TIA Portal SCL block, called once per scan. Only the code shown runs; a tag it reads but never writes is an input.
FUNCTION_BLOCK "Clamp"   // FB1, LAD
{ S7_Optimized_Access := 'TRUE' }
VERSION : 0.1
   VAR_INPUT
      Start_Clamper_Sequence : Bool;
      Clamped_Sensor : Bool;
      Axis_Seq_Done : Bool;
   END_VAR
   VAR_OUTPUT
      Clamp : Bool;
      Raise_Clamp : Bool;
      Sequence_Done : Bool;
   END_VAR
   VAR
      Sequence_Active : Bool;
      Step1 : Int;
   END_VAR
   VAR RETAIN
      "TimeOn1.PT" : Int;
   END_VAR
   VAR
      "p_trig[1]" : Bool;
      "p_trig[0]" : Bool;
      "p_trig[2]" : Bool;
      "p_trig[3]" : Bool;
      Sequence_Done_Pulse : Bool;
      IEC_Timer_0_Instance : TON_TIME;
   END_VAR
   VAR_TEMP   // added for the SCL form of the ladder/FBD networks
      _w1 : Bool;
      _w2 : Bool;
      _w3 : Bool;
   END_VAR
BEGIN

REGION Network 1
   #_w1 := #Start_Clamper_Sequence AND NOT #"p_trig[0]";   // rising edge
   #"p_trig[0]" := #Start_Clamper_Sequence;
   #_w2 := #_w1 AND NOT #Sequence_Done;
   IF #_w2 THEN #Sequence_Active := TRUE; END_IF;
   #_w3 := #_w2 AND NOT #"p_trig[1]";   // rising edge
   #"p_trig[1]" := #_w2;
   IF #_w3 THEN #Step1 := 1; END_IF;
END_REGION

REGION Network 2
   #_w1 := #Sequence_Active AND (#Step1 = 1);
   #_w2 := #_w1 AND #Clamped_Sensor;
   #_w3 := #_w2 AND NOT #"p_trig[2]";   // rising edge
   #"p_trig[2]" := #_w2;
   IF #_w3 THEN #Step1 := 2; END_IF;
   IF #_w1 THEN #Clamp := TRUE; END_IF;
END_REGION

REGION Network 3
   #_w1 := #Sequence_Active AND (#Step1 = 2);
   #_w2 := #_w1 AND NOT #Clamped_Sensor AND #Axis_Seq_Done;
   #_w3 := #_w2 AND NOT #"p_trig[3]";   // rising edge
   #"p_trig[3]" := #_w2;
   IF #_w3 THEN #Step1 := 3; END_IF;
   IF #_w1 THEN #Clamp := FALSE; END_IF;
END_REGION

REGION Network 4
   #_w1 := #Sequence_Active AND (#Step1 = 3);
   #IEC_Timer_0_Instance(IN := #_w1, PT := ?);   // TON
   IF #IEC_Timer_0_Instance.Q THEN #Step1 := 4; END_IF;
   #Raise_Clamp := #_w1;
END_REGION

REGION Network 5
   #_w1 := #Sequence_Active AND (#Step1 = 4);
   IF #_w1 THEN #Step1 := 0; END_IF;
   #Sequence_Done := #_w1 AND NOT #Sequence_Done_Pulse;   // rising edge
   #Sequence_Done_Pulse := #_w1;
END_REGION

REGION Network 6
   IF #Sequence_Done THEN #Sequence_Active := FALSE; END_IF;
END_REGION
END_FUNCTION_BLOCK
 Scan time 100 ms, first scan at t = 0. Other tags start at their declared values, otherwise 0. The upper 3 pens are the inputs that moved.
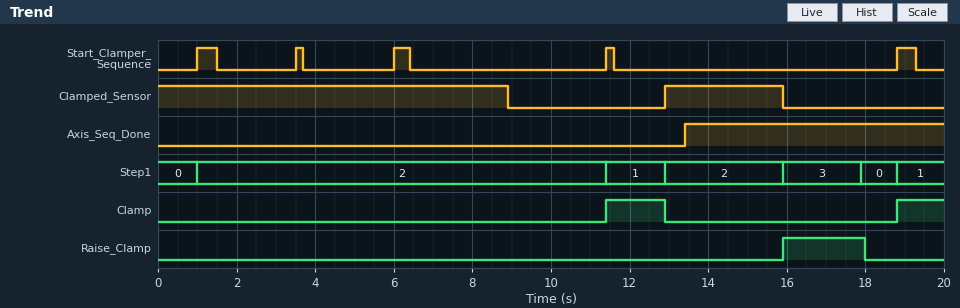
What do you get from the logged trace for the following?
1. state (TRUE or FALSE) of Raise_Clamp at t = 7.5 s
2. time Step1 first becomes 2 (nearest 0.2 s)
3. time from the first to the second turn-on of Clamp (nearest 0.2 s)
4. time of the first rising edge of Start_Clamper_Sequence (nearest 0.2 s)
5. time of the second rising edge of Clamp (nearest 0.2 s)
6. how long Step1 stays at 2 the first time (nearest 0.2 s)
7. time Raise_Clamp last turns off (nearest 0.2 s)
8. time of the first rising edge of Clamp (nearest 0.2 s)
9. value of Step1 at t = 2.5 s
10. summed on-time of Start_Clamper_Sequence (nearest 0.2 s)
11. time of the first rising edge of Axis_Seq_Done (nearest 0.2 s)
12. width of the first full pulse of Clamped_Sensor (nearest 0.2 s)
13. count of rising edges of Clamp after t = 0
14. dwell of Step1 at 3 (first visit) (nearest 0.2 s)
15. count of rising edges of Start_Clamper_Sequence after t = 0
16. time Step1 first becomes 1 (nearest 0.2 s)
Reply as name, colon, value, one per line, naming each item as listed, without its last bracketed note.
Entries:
state (TRUE or FALSE) of Raise_Clamp at t = 7.5 s: FALSE
time Step1 first becomes 2: 1.0 s
time from the first to the second turn-on of Clamp: 7.4 s
time of the first rising edge of Start_Clamper_Sequence: 1.0 s
time of the second rising edge of Clamp: 18.8 s
how long Step1 stays at 2 the first time: 10.4 s
time Raise_Clamp last turns off: 18.0 s
time of the first rising edge of Clamp: 11.4 s
value of Step1 at t = 2.5 s: 2
summed on-time of Start_Clamper_Sequence: 1.8 s
time of the first rising edge of Axis_Seq_Done: 13.4 s
width of the first full pulse of Clamped_Sensor: 3.0 s
count of rising edges of Clamp after t = 0: 2
dwell of Step1 at 3 (first visit): 2.0 s
count of rising edges of Start_Clamper_Sequence after t = 0: 5
time Step1 first becomes 1: 11.4 s
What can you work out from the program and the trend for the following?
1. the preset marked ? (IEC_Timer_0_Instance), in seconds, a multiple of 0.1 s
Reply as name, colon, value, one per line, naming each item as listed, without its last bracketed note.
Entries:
the preset marked ? (IEC_Timer_0_Instance), in seconds, a multiple of 0.1 s: 2.0 s
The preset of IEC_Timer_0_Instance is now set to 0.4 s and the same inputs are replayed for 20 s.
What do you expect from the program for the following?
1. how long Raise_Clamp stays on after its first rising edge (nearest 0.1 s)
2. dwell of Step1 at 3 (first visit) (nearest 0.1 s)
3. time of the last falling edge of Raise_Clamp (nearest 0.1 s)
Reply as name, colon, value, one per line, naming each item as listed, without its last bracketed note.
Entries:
how long Raise_Clamp stays on after its first rising edge: 0.5 s
dwell of Step1 at 3 (first visit): 0.4 s
time of the last falling edge of Raise_Clamp: 16.4 s
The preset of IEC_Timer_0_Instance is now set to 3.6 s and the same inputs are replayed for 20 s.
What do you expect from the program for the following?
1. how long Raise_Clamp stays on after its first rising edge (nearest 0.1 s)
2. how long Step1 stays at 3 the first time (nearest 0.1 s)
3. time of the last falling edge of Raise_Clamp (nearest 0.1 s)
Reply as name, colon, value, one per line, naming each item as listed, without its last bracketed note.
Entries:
how long Raise_Clamp stays on after its first rising edge: 2.9 s
how long Step1 stays at 3 the first time: 2.9 s
time of the last falling edge of Raise_Clamp: 18.8 s
